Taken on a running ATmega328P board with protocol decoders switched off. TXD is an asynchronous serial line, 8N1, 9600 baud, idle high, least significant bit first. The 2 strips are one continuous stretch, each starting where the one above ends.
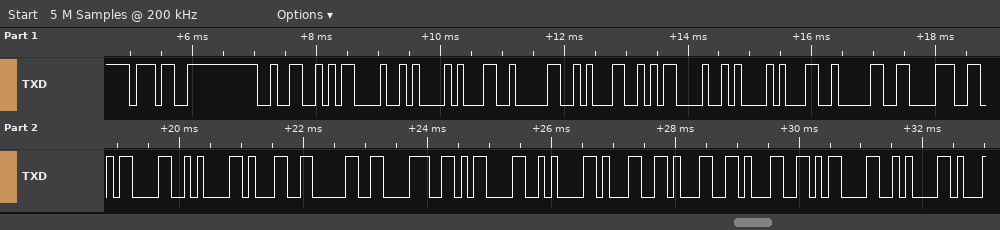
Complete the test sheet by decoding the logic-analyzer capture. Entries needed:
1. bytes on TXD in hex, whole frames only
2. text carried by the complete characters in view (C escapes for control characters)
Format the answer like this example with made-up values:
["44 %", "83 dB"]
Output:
["0x37 0x32 0x0D 0x0A 0x31 0x30 0x31 0x0D 0x0A 0x31 0x30 0x38 0x0D 0x0A 0x31 0x30 0x38 0x0D 0x0A 0x31 0x31 0x31 0x0D 0x0A", "\"72\\r\\n101\\r\\n108\\r\\n108\\r\\n111\\r\\n\""]
